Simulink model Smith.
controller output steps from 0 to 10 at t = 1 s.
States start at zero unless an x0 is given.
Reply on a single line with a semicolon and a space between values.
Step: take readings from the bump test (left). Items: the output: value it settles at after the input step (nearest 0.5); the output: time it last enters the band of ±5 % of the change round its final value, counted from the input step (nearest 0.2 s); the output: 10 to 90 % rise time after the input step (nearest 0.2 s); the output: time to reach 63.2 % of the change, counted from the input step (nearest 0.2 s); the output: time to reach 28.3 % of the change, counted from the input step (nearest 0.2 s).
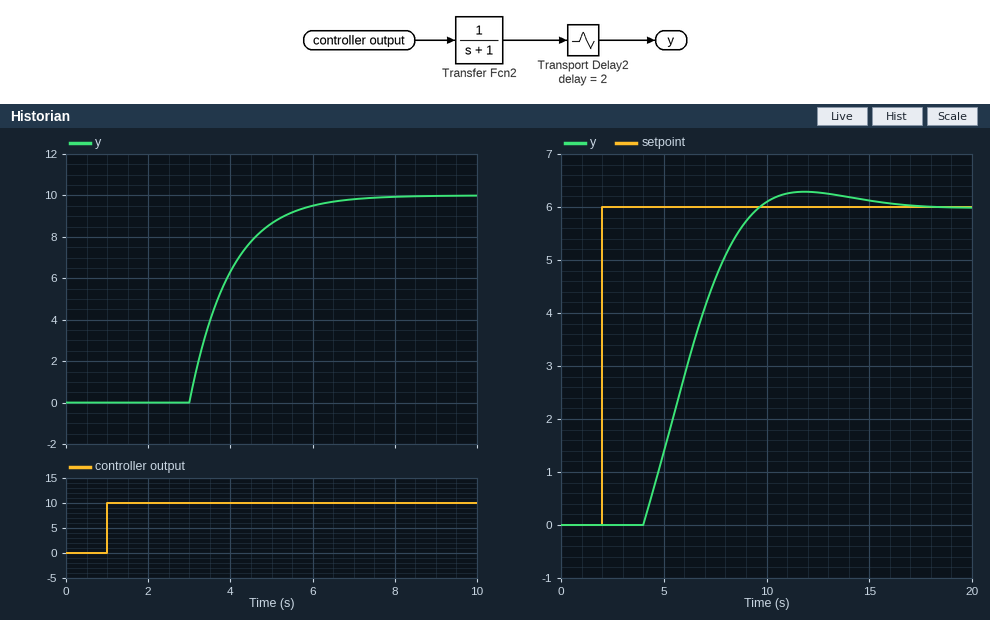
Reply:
10.0; 5.0 s; 2.2 s; 3.0 s; 2.4 s
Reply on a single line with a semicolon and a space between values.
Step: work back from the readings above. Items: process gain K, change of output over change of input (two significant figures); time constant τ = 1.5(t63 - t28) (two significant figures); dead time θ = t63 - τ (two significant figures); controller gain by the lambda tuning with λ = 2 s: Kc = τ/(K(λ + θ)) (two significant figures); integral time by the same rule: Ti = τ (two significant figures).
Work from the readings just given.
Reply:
1.0; 0.90 s; 2.1 s; 0.22; 0.90 s
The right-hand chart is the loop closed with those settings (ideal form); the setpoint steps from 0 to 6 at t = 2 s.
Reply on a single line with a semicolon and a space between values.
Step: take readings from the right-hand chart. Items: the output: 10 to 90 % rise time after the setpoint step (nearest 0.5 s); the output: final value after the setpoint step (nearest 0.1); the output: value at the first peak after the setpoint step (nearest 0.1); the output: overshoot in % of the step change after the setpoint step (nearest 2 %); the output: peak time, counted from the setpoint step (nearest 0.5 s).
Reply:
4.0 s; 6.0; 6.3; 4 %; 10.0 s
